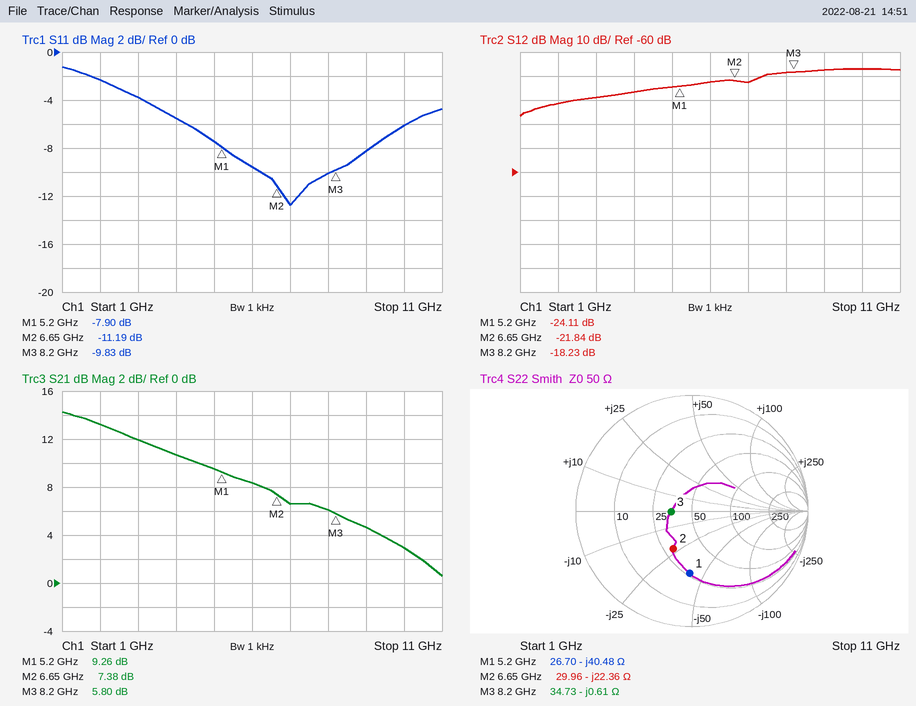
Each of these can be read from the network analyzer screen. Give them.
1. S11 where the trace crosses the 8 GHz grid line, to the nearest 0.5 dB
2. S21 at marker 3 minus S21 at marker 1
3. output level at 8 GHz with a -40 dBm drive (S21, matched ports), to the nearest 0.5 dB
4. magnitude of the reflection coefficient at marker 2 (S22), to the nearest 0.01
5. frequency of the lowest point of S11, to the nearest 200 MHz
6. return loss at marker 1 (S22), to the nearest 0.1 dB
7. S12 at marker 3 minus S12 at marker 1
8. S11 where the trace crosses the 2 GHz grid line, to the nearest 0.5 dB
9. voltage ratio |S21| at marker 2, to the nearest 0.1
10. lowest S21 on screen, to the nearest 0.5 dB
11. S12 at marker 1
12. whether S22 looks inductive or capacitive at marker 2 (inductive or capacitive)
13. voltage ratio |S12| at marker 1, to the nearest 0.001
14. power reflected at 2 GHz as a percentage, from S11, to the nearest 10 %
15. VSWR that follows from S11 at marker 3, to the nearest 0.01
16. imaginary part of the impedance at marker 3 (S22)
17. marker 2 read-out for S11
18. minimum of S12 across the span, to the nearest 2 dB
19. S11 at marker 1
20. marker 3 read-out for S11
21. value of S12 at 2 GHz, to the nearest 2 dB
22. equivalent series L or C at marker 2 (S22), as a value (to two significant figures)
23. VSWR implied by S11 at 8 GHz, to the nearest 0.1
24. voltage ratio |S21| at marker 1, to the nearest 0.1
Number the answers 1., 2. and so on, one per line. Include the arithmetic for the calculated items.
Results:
1. -10.0 dB
2. 5.8 − (9.26) = -3.46 dB
3. -40 dBm + (6.0 dB) = -34.0 dBm
4. 0.36
5. 7.0 GHz
6. 5.4 dB
7. -18.23 − (-24.11) = 5.88 dB
8. -2.5 dB
9. 10^(7.38/20) ≈ 2.3
10. 0.5 dB
11. -24.11 dB
12. capacitive
13. 10^(-24.11/20) ≈ 0.062
14. 10^(-2.5/10) ≈ 56.2 %, so 60 % to the nearest 10 %
15. (1 + 0.3225)/(1 − 0.3225) ≈ 1.95
16. -0.61 Ω
17. -11.19 dB
18. -36 dB
19. -7.90 dB
20. -9.83 dB
21. -32 dB
22. C = 1/(2π × 6.65 GHz × 22.36 Ω) ≈ 1.1 pF
23. |Γ| = 10^(-10/20) = 0.3162; VSWR = (1 + 0.3162)/(1 − 0.3162) ≈ 1.9
24. 10^(9.26/20) ≈ 2.9
